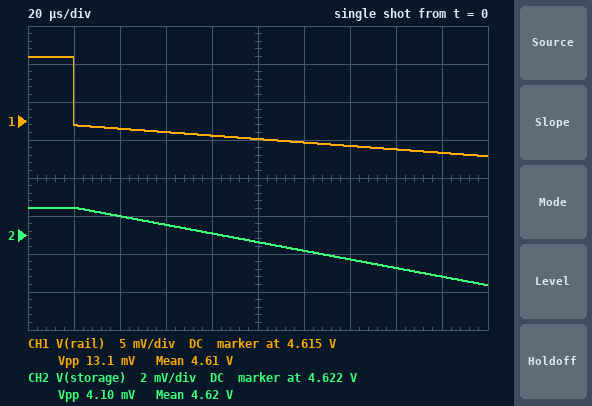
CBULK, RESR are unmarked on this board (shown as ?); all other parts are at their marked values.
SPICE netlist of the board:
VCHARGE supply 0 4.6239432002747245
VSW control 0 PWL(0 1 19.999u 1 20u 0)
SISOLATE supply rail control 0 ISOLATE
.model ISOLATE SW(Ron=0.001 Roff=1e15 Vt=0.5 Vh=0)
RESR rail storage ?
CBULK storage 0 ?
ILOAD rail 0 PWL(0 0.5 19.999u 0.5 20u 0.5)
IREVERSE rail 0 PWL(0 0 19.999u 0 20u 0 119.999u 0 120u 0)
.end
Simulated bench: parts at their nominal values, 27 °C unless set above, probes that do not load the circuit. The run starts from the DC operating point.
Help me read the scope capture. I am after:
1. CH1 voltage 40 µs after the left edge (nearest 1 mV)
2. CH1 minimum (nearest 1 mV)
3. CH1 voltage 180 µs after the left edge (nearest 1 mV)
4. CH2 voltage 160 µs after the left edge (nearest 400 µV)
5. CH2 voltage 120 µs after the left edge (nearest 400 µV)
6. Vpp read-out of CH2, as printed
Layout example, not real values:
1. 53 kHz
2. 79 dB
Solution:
1. 4.614 V
2. 4.610 V
3. 4.611 V
4. 4.6204 V
5. 4.6212 V
6. 4.10 mV
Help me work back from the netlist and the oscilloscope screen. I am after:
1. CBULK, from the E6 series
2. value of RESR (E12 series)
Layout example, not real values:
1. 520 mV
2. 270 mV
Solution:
1. 22 mF
2. 0.018 Ω
